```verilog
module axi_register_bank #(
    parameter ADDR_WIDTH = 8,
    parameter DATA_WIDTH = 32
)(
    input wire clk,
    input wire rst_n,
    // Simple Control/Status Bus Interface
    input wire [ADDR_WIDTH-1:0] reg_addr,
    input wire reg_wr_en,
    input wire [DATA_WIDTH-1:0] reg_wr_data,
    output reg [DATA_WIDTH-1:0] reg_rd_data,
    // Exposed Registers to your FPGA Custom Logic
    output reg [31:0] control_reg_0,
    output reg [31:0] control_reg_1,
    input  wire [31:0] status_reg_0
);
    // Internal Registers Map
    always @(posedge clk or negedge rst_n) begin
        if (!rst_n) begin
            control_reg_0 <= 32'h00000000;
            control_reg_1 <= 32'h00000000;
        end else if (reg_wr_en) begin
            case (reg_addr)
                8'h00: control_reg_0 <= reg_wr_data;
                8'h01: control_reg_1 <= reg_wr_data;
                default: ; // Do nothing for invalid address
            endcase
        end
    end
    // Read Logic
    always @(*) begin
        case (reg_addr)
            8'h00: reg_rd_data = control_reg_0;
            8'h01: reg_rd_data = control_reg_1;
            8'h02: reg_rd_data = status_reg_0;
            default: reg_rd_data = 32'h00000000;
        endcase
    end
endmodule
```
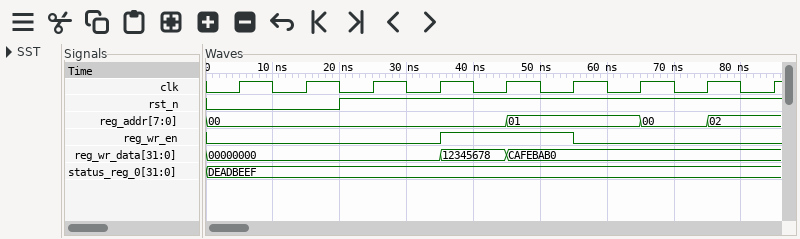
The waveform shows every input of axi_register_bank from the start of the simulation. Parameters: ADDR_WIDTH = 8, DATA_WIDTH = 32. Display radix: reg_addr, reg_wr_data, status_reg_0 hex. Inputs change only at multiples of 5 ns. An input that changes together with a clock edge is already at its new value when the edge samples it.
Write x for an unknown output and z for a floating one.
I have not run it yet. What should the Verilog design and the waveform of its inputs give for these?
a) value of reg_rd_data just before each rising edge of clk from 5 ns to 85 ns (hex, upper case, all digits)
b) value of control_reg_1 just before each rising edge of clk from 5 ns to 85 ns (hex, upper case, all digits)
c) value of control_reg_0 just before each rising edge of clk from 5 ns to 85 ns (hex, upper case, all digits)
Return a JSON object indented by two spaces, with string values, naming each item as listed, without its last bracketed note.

{
  "value of reg_rd_data just before each rising edge of clk from 5 ns to 85 ns": "00000000, 00000000, 00000000, 00000000, 12345678, CAFEBAB0, CAFEBAB0, 12345678, DEADBEEF",
  "value of control_reg_1 just before each rising edge of clk from 5 ns to 85 ns": "00000000, 00000000, 00000000, 00000000, 00000000, CAFEBAB0, CAFEBAB0, CAFEBAB0, CAFEBAB0",
  "value of control_reg_0 just before each rising edge of clk from 5 ns to 85 ns": "00000000, 00000000, 00000000, 00000000, 12345678, 12345678, 12345678, 12345678, 12345678"
}
